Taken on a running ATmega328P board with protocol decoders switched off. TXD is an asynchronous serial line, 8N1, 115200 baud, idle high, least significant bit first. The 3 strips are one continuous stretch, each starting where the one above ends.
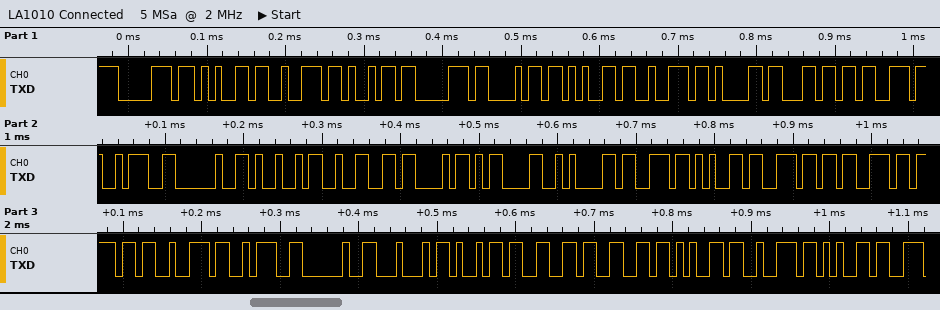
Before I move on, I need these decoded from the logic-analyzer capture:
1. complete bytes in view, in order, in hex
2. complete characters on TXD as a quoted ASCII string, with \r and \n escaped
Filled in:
70 65 72 69 70 68 65 72 61 6C 73 3A 20 49 32 43 0D 0A 73 65 6E 73 6F 72 3A 20 44 69 66 66 65 72 65
"peripherals: I2C\r\nsensor: Differe"
